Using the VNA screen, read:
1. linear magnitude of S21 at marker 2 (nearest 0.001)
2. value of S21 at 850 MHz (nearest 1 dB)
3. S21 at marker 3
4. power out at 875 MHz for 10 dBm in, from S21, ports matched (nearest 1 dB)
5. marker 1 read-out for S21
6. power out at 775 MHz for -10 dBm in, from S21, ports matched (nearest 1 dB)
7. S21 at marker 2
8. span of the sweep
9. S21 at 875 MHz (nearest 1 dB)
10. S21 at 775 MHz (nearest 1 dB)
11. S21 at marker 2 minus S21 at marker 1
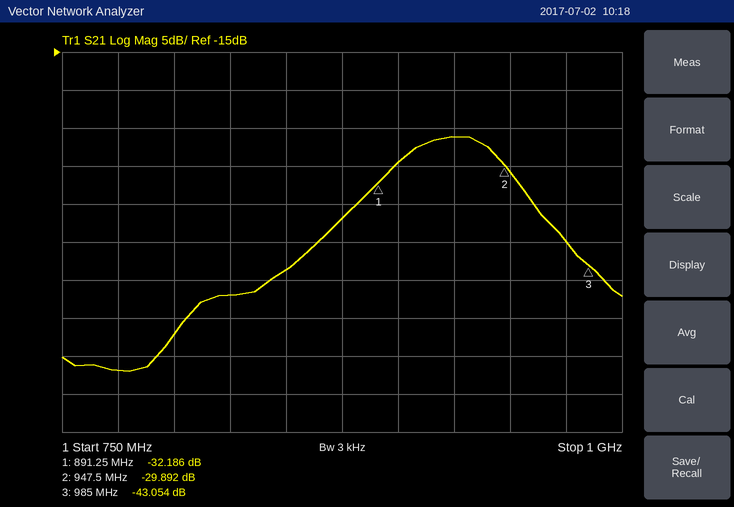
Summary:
0.032
-44 dB
-43.054 dB
-27 dBm
-32.186 dB
-67 dBm
-29.892 dB
250 MHz
-37 dB
-57 dB
2.294 dB
